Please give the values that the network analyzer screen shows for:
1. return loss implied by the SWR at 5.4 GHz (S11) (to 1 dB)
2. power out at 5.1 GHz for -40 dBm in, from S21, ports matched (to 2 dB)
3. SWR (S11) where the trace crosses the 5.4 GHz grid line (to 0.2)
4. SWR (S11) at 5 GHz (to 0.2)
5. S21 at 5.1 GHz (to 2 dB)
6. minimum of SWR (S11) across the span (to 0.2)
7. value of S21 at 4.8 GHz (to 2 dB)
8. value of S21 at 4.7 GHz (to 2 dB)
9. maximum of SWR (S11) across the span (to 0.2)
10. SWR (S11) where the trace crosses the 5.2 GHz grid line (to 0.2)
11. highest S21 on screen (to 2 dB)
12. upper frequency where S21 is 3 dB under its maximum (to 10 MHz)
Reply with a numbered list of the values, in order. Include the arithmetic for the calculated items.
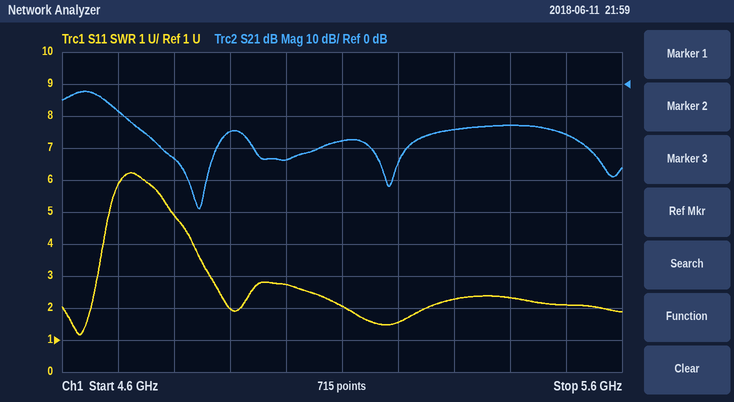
1. −20 log10((2.4 − 1)/(2.4 + 1)) ≈ 8 dB
2. -40 dBm + (-18 dB) = -58 dBm
3. 2.4
4. 2.8
5. -18 dB
6. 1.2
7. -24 dB
8. -8 dB
9. 6.2
10. 1.6
11. -2 dB
12. 4.68 GHz
